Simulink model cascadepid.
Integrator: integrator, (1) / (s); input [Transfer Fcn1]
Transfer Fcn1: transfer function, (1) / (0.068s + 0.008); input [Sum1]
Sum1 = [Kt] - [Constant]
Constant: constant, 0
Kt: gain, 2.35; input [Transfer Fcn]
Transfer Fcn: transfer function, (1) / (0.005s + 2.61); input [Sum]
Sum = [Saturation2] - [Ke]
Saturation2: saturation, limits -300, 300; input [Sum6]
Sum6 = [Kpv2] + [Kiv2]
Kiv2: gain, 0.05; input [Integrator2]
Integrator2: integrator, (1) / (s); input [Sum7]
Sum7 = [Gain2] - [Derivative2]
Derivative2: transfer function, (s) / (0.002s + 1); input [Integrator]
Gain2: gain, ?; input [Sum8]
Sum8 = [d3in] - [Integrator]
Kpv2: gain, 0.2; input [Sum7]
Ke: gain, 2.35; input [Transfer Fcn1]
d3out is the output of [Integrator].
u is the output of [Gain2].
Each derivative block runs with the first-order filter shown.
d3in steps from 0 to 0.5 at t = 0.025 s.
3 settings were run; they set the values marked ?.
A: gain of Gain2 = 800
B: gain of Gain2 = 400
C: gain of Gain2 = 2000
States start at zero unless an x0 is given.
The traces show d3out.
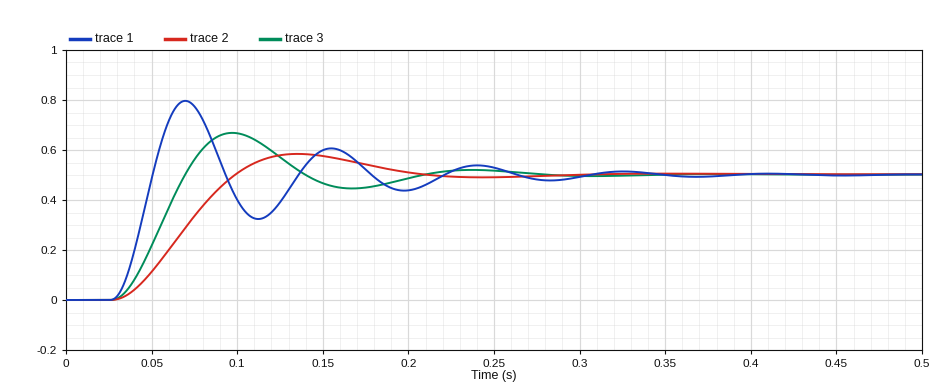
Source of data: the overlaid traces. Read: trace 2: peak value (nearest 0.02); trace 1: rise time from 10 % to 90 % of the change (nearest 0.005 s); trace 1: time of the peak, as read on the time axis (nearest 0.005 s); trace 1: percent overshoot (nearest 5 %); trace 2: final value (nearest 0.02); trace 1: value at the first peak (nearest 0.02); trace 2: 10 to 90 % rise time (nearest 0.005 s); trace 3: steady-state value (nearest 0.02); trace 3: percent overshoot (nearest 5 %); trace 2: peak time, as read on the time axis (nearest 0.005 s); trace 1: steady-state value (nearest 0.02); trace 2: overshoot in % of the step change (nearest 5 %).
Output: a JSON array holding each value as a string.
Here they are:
["0.58", "0.015 s", "0.070 s", "60 %", "0.50", "0.80", "0.050 s", "0.50", "35 %", "0.135 s", "0.50", "15 %"]
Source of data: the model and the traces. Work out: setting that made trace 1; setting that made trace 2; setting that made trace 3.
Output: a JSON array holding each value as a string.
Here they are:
["C", "B", "A"]
